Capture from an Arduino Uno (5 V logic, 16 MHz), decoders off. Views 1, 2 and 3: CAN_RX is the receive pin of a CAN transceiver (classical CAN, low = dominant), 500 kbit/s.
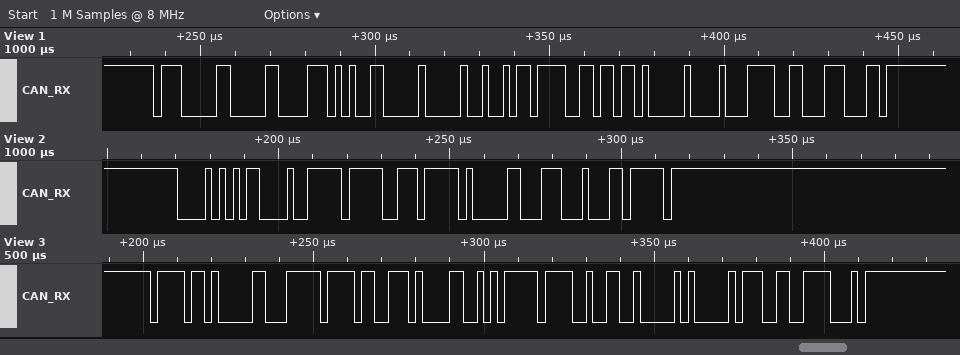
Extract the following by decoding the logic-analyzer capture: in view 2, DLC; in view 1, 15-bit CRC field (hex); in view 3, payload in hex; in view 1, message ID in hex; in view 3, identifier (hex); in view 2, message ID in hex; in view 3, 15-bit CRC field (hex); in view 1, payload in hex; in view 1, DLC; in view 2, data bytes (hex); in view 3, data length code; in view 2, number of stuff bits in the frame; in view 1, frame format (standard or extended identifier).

4
0x4C71
FF B3 A1 95 FF 26 40 81
0x704
0x7B4
0x0AB
0x6678
75 30 00 96 F3 6D 00 47
8
FF DD F8 23
8
4
standard
